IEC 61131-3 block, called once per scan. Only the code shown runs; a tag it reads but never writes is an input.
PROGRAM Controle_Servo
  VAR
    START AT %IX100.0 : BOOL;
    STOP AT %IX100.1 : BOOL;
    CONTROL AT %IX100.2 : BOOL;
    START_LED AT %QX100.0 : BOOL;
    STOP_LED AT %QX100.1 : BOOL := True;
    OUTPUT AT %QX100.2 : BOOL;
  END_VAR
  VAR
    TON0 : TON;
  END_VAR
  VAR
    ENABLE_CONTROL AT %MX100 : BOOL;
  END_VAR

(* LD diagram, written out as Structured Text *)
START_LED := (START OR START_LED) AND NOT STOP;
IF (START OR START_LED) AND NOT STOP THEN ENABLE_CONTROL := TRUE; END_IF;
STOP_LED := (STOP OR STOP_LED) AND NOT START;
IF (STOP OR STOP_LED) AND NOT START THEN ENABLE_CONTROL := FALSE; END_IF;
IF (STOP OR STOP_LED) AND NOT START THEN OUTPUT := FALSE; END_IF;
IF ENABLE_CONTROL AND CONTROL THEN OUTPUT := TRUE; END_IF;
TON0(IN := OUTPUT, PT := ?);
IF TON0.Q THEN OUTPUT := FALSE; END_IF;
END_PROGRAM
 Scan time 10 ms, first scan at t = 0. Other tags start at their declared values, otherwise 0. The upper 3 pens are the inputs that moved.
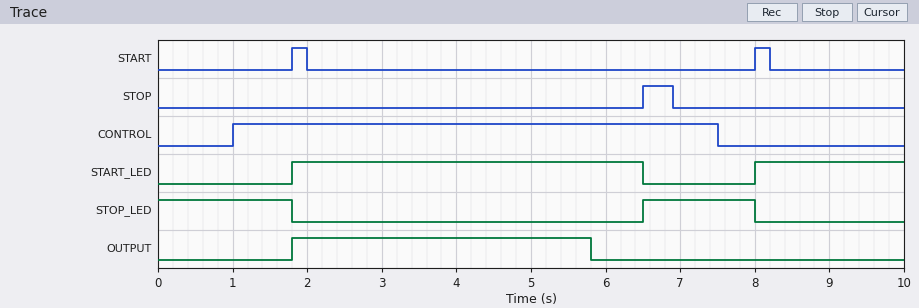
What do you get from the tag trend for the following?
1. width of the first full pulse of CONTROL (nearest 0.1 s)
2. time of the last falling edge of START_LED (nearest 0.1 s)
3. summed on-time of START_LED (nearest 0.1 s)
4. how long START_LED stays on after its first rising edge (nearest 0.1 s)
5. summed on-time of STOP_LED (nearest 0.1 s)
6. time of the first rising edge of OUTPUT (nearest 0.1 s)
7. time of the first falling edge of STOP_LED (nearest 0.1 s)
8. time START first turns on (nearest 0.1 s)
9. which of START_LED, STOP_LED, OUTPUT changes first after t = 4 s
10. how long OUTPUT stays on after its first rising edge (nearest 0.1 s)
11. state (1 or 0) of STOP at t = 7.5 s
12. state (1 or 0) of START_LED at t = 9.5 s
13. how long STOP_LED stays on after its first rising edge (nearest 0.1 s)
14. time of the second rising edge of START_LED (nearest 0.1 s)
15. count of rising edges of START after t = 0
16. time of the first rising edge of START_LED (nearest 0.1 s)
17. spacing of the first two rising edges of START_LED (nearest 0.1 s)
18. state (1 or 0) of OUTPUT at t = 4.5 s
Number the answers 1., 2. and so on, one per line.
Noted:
1. 6.5 s
2. 6.5 s
3. 6.7 s
4. 4.7 s
5. 3.3 s
6. 1.8 s
7. 1.8 s
8. 1.8 s
9. OUTPUT
10. 4.0 s
11. 0
12. 1
13. 1.5 s
14. 8.0 s
15. 2
16. 1.8 s
17. 6.2 s
18. 1
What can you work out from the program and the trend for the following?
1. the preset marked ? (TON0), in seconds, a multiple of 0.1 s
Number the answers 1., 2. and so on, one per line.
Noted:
1. 4.0 s
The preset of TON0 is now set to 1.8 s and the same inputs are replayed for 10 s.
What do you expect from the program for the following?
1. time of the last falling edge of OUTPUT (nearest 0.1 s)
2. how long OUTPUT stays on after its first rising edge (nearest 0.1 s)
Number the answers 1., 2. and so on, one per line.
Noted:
1. 3.6 s
2. 1.8 s
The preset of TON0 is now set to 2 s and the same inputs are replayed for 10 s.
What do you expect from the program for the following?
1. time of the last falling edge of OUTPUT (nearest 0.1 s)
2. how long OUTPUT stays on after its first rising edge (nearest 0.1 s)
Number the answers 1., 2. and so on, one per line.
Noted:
1. 3.8 s
2. 2.0 s
